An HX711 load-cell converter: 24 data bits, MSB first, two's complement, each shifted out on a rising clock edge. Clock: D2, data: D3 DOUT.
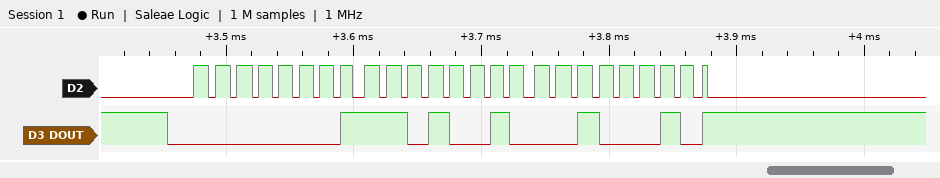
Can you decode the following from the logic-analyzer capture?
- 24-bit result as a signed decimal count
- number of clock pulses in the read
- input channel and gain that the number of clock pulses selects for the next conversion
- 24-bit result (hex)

119330
25
channel A, gain 128
0x01D222
